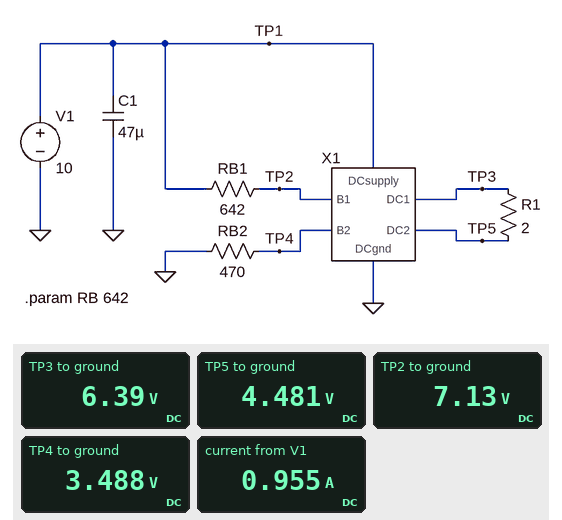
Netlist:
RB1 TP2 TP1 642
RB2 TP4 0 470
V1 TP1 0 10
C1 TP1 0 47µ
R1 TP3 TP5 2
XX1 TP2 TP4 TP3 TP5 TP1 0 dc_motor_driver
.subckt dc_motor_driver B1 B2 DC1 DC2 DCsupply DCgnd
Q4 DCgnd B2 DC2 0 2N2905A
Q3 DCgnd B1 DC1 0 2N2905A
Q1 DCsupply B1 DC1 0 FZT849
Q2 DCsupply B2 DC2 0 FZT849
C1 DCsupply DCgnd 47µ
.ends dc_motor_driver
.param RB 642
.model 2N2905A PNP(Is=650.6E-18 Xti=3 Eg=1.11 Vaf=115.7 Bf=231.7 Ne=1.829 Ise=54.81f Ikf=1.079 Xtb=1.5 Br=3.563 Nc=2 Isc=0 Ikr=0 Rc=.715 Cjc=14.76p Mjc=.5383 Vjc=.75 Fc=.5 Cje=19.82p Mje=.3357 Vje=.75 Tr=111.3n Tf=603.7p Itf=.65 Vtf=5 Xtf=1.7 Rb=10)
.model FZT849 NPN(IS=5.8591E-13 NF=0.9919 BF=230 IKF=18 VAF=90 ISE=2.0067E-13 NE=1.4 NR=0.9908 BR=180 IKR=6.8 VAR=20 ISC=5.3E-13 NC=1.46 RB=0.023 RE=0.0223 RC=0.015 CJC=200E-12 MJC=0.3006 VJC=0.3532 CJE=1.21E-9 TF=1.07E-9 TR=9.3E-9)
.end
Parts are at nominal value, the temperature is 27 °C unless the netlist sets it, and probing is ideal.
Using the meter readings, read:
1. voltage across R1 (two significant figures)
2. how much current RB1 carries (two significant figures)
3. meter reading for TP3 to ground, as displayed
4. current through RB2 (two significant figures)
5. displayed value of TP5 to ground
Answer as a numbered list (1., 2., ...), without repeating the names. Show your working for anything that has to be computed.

1. 6.39 V - 4.481 V = 1.9 V
2. (10 V - 7.13 V) / 642 Ω = 4.5 mA
3. 6.39 V
4. (3.488 V) / 470 Ω = 7.4 mA
5. 4.481 V
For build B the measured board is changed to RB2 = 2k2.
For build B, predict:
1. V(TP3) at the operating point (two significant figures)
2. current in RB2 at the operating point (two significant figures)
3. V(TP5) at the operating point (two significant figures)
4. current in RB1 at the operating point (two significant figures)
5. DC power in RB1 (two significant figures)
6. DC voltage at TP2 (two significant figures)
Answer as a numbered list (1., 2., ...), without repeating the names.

1. 7.9 V
2. 2.7 mA
3. 6.9 V
4. 2.2 mA
5. 3.1 mW
6. 8.6 V
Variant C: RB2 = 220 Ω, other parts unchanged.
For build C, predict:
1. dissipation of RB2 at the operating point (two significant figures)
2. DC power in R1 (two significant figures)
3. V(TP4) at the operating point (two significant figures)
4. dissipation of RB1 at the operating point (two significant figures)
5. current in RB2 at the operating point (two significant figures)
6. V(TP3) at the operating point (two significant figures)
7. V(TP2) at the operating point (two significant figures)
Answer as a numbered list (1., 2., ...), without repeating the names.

1. 24 mW
2. 2.8 W
3. 2.3 V
4. 20 mW
5. 10 mA
6. 5.7 V
7. 6.4 V
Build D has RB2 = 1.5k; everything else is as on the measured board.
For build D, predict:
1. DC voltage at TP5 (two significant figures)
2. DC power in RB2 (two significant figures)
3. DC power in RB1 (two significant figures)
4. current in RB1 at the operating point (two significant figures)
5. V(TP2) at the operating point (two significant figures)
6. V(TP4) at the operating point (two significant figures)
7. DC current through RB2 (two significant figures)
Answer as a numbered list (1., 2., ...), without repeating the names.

1. 6.4 V
2. 20 mW
3. 4.7 mW
4. 2.7 mA
5. 8.3 V
6. 5.4 V
7. 3.6 mA
